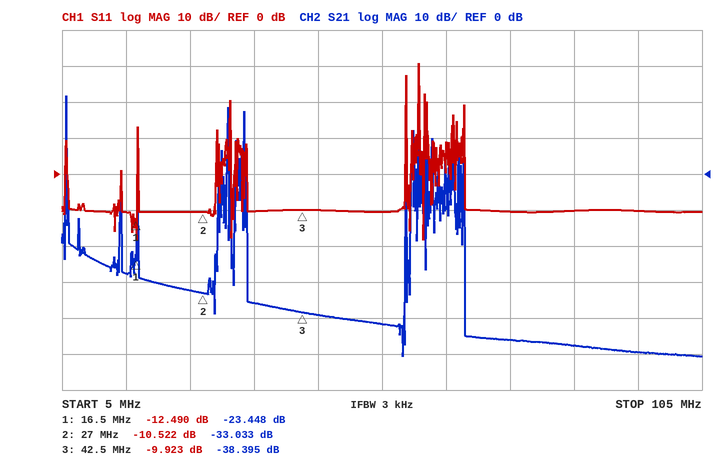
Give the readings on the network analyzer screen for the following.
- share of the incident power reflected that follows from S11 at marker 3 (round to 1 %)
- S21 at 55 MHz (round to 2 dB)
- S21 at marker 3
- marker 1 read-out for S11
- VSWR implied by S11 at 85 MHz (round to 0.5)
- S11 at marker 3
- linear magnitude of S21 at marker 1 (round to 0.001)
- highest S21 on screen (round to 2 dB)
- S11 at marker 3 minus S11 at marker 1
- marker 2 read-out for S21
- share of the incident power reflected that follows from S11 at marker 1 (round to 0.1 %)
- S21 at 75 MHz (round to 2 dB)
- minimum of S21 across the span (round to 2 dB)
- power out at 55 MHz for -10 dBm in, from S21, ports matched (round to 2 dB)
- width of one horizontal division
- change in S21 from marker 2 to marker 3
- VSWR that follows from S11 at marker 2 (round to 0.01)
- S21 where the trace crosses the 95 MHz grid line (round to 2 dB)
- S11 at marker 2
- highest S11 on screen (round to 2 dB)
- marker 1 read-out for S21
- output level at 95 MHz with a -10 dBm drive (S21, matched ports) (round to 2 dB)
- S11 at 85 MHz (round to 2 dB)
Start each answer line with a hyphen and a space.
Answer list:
- 10 %
- -42 dB
- -38.395 dB
- -12.490 dB
- 2.0
- -9.923 dB
- 0.067
- 22 dB
- 2.567 dB
- -33.033 dB
- 5.6 %
- -46 dB
- -50 dB
- -52 dBm
- 10 MHz
- -5.362 dB
- 1.85
- -50 dB
- -10.522 dB
- 30 dB
- -23.448 dB
- -60 dBm
- -10 dB
